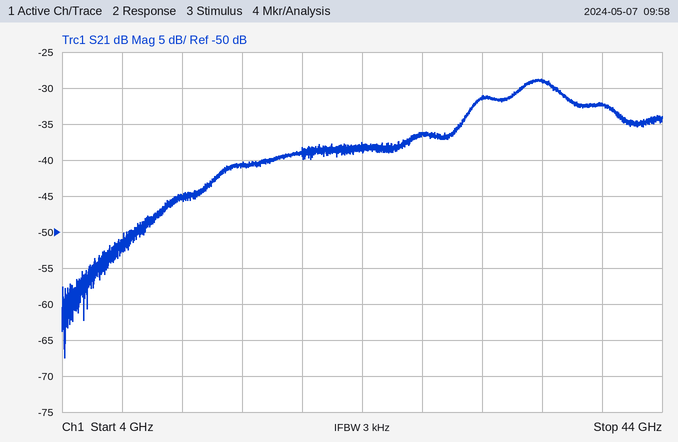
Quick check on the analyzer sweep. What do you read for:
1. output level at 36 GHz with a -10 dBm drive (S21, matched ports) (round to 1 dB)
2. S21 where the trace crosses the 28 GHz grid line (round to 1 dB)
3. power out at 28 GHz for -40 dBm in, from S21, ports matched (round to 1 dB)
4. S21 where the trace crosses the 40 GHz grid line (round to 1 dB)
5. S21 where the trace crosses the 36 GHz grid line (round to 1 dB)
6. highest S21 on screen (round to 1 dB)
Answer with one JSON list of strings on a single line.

["-39 dBm", "-36 dB", "-76 dBm", "-32 dB", "-29 dB", "-29 dB"]
